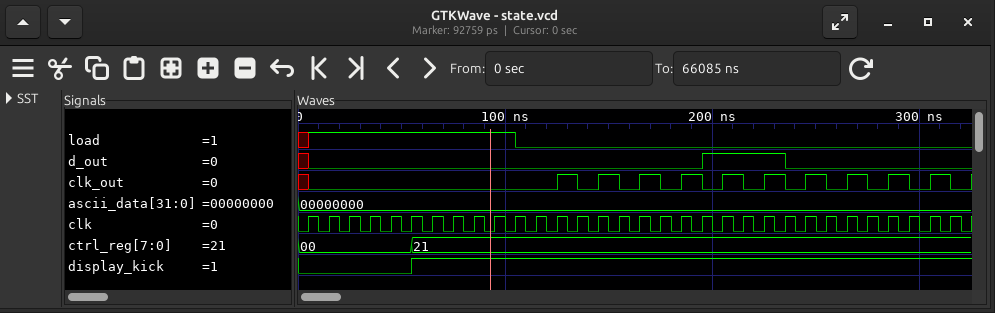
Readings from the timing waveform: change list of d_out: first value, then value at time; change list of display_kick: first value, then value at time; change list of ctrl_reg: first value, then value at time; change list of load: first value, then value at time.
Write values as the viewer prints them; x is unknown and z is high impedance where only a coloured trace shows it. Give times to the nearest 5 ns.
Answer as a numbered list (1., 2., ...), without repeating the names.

1. x, 0 at 5 ns, 1 at 195 ns, 0 at 235 ns
2. 0, 1 at 55 ns
3. 00, 21 at 55 ns
4. x, 1 at 5 ns, 0 at 105 ns
